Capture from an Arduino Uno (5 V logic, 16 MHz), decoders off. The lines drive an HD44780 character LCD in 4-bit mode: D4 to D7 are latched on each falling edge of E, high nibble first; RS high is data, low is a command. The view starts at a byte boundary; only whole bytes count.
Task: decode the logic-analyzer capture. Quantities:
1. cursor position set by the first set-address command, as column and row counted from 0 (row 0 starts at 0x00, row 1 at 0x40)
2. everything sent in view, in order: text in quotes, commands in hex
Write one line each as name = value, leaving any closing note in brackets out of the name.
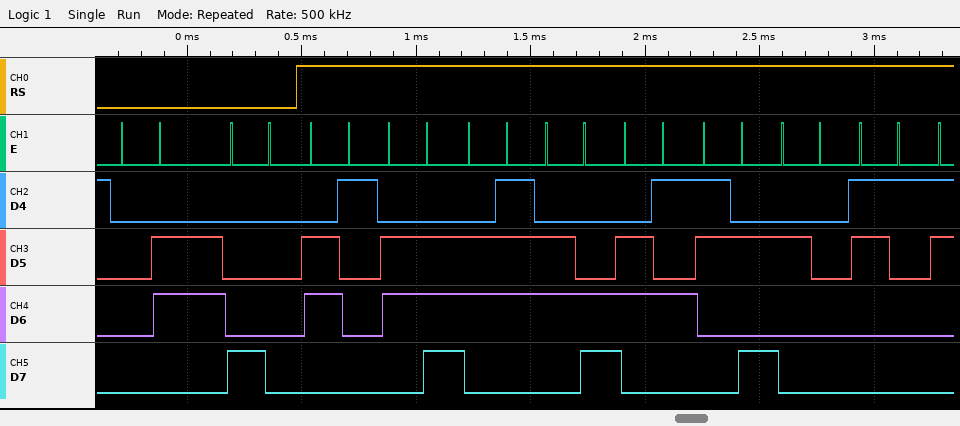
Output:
cursor position set by the first set-address command, as column and row counted from 0 = column 0, row 0
everything sent in view, in order: text in quotes, commands in hex = 0x06 0x80 "angle: 1"
